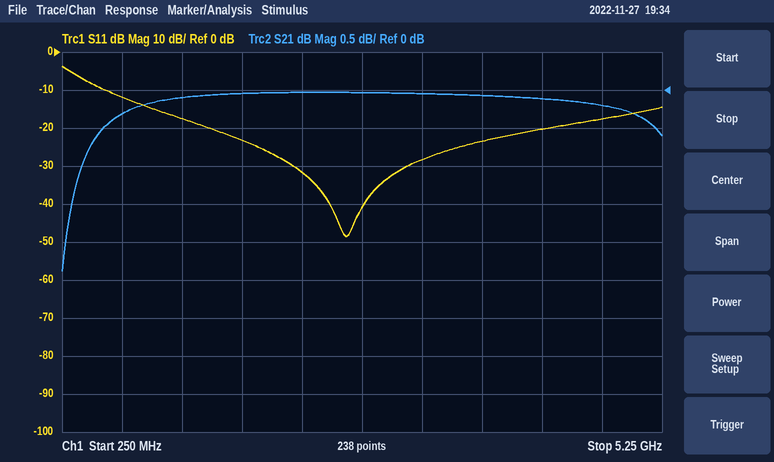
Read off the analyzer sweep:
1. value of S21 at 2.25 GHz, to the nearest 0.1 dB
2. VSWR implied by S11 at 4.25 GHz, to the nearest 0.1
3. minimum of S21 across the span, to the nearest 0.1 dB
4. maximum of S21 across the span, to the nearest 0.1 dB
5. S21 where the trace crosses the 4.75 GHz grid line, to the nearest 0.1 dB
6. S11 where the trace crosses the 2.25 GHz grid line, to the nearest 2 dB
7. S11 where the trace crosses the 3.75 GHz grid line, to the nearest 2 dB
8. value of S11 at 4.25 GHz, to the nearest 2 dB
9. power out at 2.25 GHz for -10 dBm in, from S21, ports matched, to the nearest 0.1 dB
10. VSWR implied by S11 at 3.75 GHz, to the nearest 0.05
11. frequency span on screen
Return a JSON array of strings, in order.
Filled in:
["0.0 dB", "1.2", "-2.4 dB", "0.0 dB", "-0.2 dB", "-32 dB", "-24 dB", "-20 dB", "-10.0 dBm", "1.15", "5 GHz"]
